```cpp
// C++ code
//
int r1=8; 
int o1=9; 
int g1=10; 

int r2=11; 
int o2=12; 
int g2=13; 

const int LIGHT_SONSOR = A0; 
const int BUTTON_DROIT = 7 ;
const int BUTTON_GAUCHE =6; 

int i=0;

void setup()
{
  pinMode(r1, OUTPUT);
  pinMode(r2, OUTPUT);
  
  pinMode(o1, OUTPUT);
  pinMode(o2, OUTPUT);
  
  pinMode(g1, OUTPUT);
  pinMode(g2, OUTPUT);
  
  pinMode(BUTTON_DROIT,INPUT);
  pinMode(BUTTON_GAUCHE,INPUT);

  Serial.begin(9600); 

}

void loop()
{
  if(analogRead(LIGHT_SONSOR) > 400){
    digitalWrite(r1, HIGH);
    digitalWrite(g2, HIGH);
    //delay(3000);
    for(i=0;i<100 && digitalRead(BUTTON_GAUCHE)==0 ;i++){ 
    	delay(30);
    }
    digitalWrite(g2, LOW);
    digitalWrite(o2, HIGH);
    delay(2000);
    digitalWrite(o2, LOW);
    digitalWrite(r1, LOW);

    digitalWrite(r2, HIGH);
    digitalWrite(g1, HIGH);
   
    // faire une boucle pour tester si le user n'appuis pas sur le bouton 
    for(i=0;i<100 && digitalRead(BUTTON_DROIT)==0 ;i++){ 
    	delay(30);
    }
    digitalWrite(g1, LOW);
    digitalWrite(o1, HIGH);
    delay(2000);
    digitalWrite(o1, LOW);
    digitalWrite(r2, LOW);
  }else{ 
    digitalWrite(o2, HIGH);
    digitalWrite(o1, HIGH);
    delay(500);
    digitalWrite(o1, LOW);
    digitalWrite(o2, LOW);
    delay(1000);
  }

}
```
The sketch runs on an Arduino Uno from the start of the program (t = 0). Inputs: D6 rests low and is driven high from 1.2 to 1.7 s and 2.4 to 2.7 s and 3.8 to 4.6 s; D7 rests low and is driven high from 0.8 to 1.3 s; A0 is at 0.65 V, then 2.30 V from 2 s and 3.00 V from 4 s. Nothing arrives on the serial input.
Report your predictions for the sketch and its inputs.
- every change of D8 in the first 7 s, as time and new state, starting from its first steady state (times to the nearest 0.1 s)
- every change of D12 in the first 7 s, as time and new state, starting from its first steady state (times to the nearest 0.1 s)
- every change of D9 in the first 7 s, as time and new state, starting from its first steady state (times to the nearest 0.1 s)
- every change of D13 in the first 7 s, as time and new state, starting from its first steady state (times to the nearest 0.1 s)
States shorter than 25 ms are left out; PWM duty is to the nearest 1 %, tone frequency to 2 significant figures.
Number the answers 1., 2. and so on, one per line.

1. 0 s low; 3 s high; 5.8 s low
2. 0 s high; 0.5 s low; 1.5 s high; 2 s low; 3.8 s high; 5.8 s low
3. 0 s high; 0.5 s low; 1.5 s high; 2 s low
4. 0 s low; 3 s high; 3.8 s low
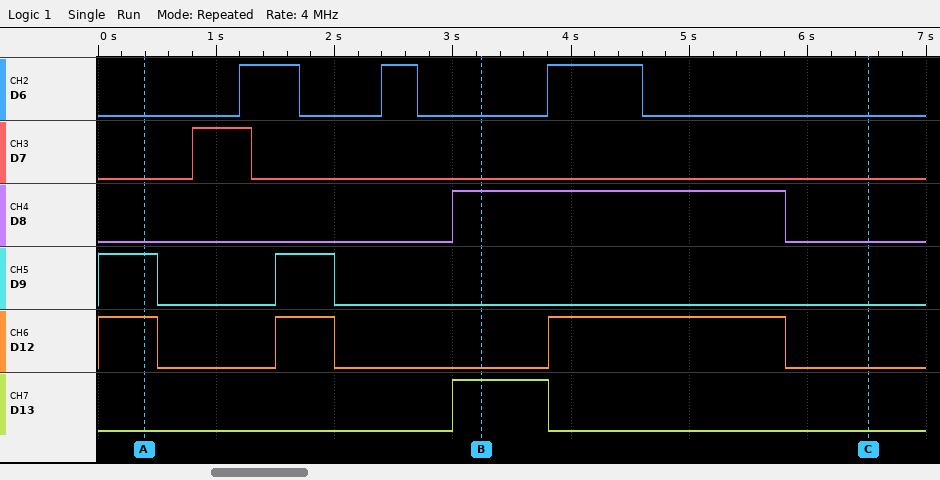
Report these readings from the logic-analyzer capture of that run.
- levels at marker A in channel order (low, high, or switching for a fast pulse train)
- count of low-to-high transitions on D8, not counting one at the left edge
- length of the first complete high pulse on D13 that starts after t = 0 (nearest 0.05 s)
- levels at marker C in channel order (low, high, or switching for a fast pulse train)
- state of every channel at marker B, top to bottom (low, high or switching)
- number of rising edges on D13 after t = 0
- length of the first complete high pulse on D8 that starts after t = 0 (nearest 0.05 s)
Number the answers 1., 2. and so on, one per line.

1. D6 low, D7 low, D8 low, D9 high, D12 high, D13 low
2. 1
3. 0.80 s
4. D6 low, D7 low, D8 low, D9 low, D12 low, D13 low
5. D6 low, D7 low, D8 high, D9 low, D12 low, D13 high
6. 1
7. 2.80 s
